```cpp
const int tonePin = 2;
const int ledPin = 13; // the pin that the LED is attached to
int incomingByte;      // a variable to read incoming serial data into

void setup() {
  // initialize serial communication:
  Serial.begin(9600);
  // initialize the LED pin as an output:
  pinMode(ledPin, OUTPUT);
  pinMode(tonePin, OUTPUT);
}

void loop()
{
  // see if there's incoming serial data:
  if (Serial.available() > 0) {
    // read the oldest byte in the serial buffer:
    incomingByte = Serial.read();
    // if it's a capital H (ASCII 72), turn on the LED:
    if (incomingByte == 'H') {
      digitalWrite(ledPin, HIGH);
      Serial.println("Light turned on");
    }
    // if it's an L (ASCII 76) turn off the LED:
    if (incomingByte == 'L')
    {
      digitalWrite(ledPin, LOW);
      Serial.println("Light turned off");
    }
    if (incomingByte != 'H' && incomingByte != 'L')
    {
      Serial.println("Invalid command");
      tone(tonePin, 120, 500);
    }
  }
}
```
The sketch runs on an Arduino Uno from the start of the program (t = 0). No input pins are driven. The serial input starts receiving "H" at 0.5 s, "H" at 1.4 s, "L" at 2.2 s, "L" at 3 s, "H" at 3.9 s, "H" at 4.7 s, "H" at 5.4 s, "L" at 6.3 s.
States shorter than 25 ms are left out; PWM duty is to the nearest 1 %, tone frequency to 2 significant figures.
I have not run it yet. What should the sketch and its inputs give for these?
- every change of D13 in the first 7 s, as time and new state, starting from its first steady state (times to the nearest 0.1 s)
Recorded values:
0 s low; 0.5 s high; 2.2 s low; 3.9 s high; 6.3 s low
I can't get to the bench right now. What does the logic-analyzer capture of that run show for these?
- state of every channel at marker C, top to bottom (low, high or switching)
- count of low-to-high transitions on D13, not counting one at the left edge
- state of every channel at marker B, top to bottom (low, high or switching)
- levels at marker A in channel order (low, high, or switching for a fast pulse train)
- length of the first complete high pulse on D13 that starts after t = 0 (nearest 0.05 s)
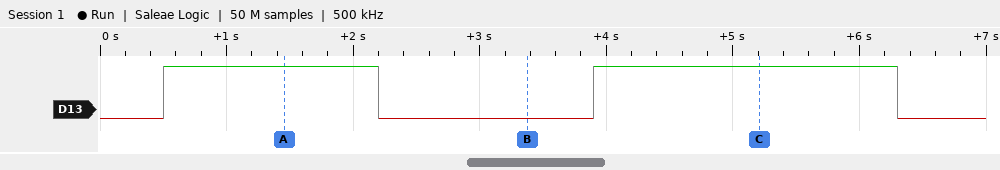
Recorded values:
D13 high
2
D13 low
D13 high
1.70 s
